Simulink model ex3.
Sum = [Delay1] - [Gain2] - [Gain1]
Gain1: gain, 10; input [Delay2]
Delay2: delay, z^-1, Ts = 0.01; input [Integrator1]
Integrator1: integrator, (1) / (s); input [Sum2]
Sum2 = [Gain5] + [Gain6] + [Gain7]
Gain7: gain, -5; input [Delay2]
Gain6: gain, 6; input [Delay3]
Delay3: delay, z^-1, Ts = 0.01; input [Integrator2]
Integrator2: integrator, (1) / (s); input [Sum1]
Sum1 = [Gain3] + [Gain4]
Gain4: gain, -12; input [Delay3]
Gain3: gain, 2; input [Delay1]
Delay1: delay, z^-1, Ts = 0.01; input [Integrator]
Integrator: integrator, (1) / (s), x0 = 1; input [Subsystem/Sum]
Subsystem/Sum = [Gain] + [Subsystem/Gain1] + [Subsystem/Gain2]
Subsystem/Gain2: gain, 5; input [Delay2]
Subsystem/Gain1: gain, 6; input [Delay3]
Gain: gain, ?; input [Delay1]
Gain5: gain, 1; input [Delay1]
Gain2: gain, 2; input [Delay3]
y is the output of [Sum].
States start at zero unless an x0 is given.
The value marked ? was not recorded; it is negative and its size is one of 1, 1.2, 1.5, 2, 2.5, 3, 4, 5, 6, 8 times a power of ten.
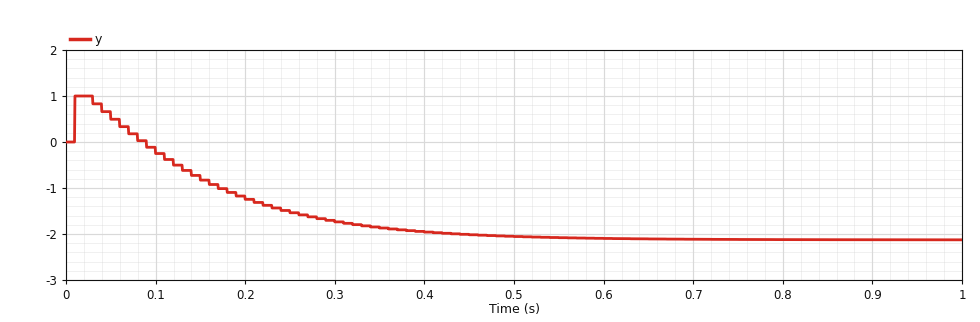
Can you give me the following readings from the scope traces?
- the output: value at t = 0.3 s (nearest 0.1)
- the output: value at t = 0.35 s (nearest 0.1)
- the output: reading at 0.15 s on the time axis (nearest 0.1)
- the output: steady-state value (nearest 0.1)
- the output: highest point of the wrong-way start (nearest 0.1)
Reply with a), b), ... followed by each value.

a) -1.7
b) -1.9
c) -0.8
d) -2.1
e) 1.0
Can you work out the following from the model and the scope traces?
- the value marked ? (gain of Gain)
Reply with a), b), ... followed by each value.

a) -3
